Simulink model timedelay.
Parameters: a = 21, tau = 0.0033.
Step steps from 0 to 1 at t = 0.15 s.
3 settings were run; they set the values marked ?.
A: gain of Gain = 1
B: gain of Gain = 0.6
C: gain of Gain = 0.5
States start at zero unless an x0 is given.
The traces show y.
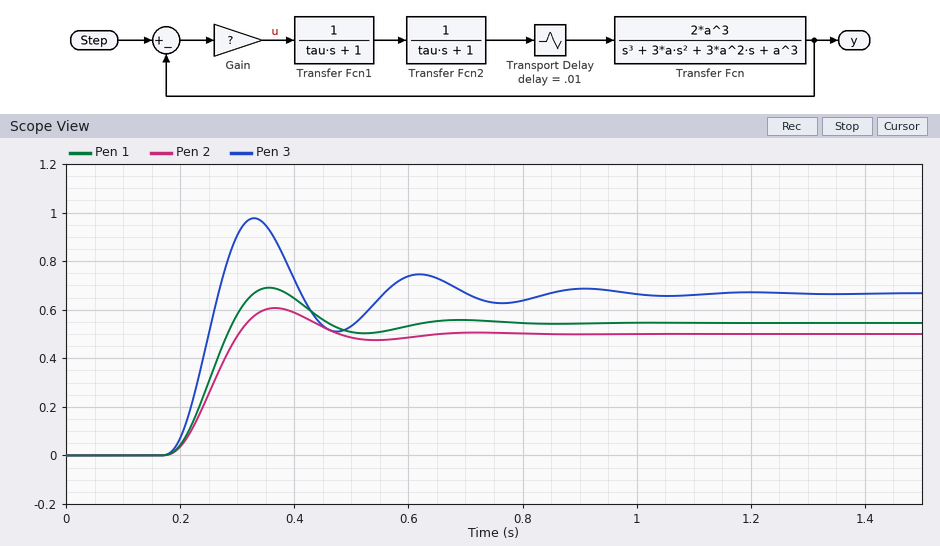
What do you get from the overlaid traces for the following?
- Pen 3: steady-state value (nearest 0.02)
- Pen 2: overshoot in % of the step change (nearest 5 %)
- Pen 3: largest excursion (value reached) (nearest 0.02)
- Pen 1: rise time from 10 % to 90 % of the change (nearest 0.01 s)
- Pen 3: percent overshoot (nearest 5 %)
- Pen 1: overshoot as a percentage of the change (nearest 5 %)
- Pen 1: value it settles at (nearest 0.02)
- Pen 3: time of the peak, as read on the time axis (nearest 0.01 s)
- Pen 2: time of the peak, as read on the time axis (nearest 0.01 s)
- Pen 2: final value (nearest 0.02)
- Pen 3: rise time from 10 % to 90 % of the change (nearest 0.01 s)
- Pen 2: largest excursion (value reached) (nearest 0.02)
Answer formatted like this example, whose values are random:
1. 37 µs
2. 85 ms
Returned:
1. 0.66
2. 20 %
3. 0.98
4. 0.08 s
5. 45 %
6. 25 %
7. 0.54
8. 0.33 s
9. 0.37 s
10. 0.50
11. 0.06 s
12. 0.60
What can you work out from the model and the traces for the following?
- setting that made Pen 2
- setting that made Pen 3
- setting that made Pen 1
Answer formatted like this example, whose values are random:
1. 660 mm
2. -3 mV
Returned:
1. C
2. A
3. B
